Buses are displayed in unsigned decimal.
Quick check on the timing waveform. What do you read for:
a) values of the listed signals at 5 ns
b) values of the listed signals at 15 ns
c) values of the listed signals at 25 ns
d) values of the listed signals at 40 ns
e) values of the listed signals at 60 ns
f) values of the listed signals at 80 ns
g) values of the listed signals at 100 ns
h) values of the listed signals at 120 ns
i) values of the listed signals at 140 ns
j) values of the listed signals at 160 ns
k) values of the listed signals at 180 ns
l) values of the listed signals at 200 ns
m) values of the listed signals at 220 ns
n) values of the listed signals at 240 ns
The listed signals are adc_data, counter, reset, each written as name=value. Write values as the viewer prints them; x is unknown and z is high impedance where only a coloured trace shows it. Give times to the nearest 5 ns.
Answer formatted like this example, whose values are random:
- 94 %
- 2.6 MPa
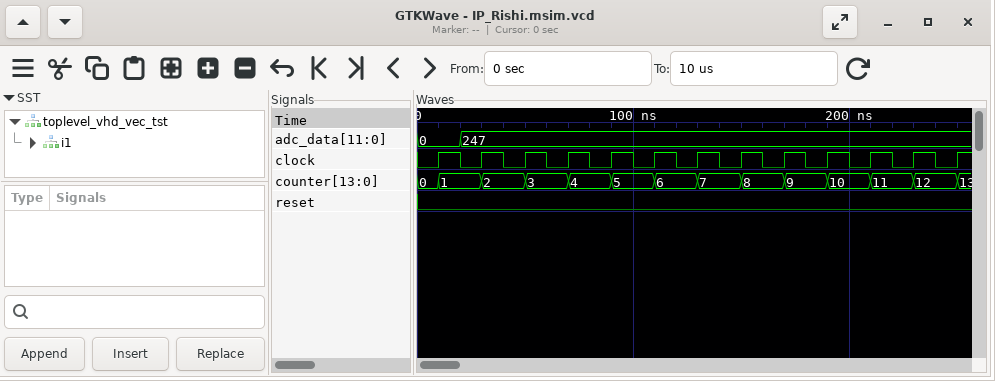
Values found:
- adc_data=0, counter=0, reset=0
- adc_data=0, counter=1, reset=0
- adc_data=247, counter=1, reset=0
- adc_data=247, counter=2, reset=0
- adc_data=247, counter=3, reset=0
- adc_data=247, counter=4, reset=0
- adc_data=247, counter=5, reset=0
- adc_data=247, counter=6, reset=0
- adc_data=247, counter=7, reset=0
- adc_data=247, counter=8, reset=0
- adc_data=247, counter=9, reset=0
- adc_data=247, counter=10, reset=0
- adc_data=247, counter=11, reset=0
- adc_data=247, counter=12, reset=0
